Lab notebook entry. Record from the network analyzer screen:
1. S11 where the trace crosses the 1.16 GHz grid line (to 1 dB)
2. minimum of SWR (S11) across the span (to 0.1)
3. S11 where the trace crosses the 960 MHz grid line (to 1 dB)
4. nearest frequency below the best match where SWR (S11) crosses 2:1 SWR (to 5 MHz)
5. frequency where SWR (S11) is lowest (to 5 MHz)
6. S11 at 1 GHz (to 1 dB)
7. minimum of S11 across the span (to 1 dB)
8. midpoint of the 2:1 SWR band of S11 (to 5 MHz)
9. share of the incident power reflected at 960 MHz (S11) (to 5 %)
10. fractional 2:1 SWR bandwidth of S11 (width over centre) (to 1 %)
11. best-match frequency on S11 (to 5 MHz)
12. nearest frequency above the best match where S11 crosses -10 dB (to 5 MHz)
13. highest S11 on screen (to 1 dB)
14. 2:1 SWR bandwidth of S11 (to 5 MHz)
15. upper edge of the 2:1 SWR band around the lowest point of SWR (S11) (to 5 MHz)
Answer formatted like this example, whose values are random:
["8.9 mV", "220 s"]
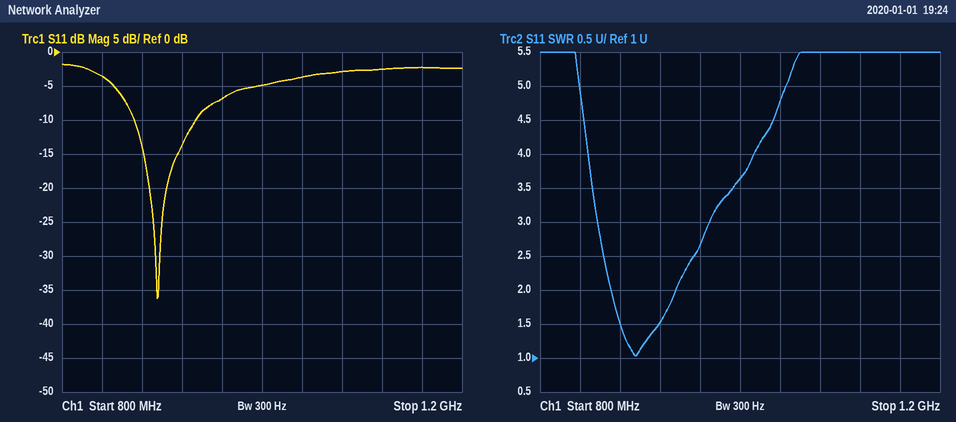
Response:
["-2 dB", "1.0", "-7 dB", "870 MHz", "895 MHz", "-5 dB", "-36 dB", "905 MHz", "20 %", "7 %", "895 MHz", "935 MHz", "-2 dB", "65 MHz", "935 MHz"]
